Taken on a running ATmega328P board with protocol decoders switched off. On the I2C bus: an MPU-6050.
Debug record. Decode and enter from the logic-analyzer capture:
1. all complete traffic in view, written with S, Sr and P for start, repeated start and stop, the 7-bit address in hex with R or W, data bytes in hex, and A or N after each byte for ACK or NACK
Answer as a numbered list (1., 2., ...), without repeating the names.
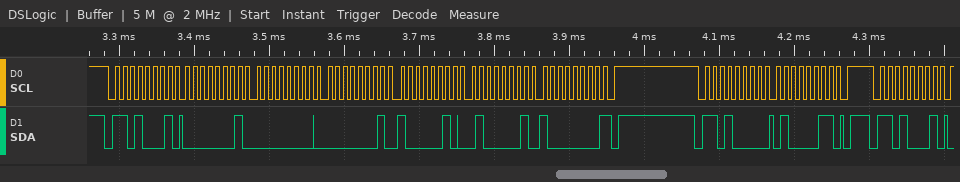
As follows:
1. S 68R A 01 A 00 A 01 A 82 A 41 A 80 N P S 68W A 43 A P S 68R A
